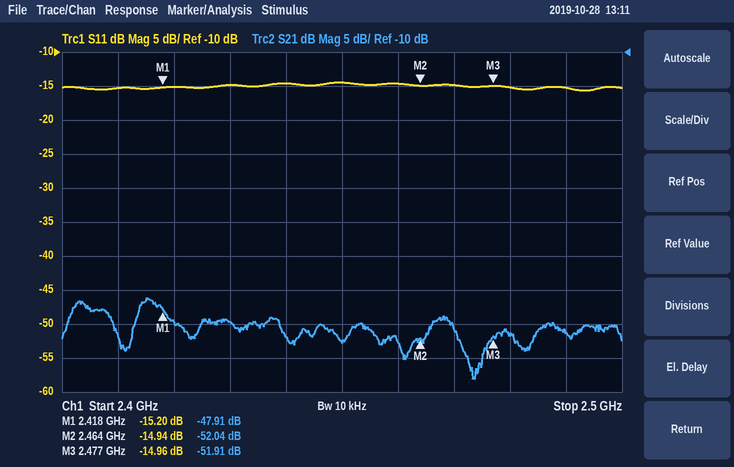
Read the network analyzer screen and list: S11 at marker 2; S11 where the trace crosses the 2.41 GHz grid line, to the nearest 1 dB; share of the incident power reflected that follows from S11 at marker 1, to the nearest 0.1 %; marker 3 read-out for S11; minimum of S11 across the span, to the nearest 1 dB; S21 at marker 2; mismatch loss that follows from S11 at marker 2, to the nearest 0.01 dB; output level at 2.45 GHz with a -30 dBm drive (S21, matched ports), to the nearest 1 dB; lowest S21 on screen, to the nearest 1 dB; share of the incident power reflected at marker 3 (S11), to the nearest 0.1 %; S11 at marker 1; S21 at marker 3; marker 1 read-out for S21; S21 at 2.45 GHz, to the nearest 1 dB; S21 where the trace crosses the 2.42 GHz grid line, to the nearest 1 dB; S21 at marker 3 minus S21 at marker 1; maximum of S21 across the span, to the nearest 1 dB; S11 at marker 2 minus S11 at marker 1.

-14.94 dB
-15 dB
3.0 %
-14.96 dB
-16 dB
-52.04 dB
0.14 dB
-83 dBm
-58 dB
3.2 %
-15.20 dB
-51.91 dB
-47.91 dB
-53 dB
-50 dB
-4.00 dB
-46 dB
0.26 dB
